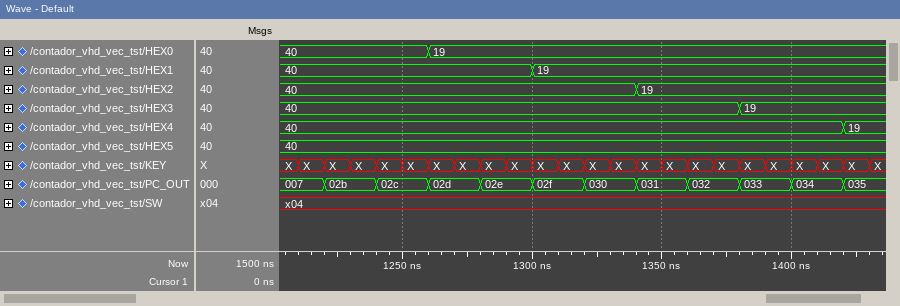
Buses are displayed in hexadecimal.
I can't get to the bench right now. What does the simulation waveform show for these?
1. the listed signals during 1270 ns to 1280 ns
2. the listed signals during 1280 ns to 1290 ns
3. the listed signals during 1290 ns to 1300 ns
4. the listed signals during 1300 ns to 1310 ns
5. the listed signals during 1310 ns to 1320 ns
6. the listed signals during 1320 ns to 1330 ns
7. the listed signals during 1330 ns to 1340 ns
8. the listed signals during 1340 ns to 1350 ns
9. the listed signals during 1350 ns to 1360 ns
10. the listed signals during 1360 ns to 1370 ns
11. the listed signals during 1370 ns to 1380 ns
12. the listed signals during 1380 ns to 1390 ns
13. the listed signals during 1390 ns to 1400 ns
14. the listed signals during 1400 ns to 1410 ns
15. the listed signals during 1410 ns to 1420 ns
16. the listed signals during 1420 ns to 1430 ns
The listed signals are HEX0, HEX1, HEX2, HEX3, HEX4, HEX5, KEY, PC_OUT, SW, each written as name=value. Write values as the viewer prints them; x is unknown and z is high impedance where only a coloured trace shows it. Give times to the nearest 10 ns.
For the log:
HEX0=19, HEX1=40, HEX2=40, HEX3=40, HEX4=40, HEX5=40, KEY=X, PC_OUT=02d, SW=x04
HEX0=19, HEX1=40, HEX2=40, HEX3=40, HEX4=40, HEX5=40, KEY=X, PC_OUT=02e, SW=x04
HEX0=19, HEX1=40, HEX2=40, HEX3=40, HEX4=40, HEX5=40, KEY=X, PC_OUT=02e, SW=x04
HEX0=19, HEX1=19, HEX2=40, HEX3=40, HEX4=40, HEX5=40, KEY=X, PC_OUT=02f, SW=x04
HEX0=19, HEX1=19, HEX2=40, HEX3=40, HEX4=40, HEX5=40, KEY=X, PC_OUT=02f, SW=x04
HEX0=19, HEX1=19, HEX2=40, HEX3=40, HEX4=40, HEX5=40, KEY=X, PC_OUT=030, SW=x04
HEX0=19, HEX1=19, HEX2=40, HEX3=40, HEX4=40, HEX5=40, KEY=X, PC_OUT=030, SW=x04
HEX0=19, HEX1=19, HEX2=19, HEX3=40, HEX4=40, HEX5=40, KEY=X, PC_OUT=031, SW=x04
HEX0=19, HEX1=19, HEX2=19, HEX3=40, HEX4=40, HEX5=40, KEY=X, PC_OUT=031, SW=x04
HEX0=19, HEX1=19, HEX2=19, HEX3=40, HEX4=40, HEX5=40, KEY=X, PC_OUT=032, SW=x04
HEX0=19, HEX1=19, HEX2=19, HEX3=40, HEX4=40, HEX5=40, KEY=X, PC_OUT=032, SW=x04
HEX0=19, HEX1=19, HEX2=19, HEX3=19, HEX4=40, HEX5=40, KEY=X, PC_OUT=033, SW=x04
HEX0=19, HEX1=19, HEX2=19, HEX3=19, HEX4=40, HEX5=40, KEY=X, PC_OUT=033, SW=x04
HEX0=19, HEX1=19, HEX2=19, HEX3=19, HEX4=40, HEX5=40, KEY=X, PC_OUT=034, SW=x04
HEX0=19, HEX1=19, HEX2=19, HEX3=19, HEX4=40, HEX5=40, KEY=X, PC_OUT=034, SW=x04
HEX0=19, HEX1=19, HEX2=19, HEX3=19, HEX4=19, HEX5=40, KEY=X, PC_OUT=035, SW=x04
